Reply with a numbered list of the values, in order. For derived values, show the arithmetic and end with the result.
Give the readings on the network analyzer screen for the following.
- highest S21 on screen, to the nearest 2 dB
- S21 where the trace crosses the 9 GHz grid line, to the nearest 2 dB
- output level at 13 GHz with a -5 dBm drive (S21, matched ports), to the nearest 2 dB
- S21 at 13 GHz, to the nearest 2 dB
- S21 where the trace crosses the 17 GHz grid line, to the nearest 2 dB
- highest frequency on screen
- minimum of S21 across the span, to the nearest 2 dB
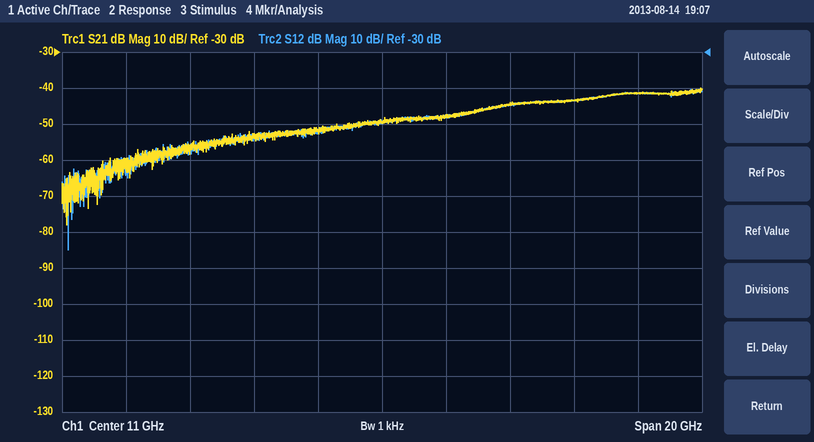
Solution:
1. -40 dB
2. -52 dB
3. -5 dBm + (-48 dB) = -52 dBm
4. -48 dB
5. -44 dB
6. 21 GHz
7. -78 dB
